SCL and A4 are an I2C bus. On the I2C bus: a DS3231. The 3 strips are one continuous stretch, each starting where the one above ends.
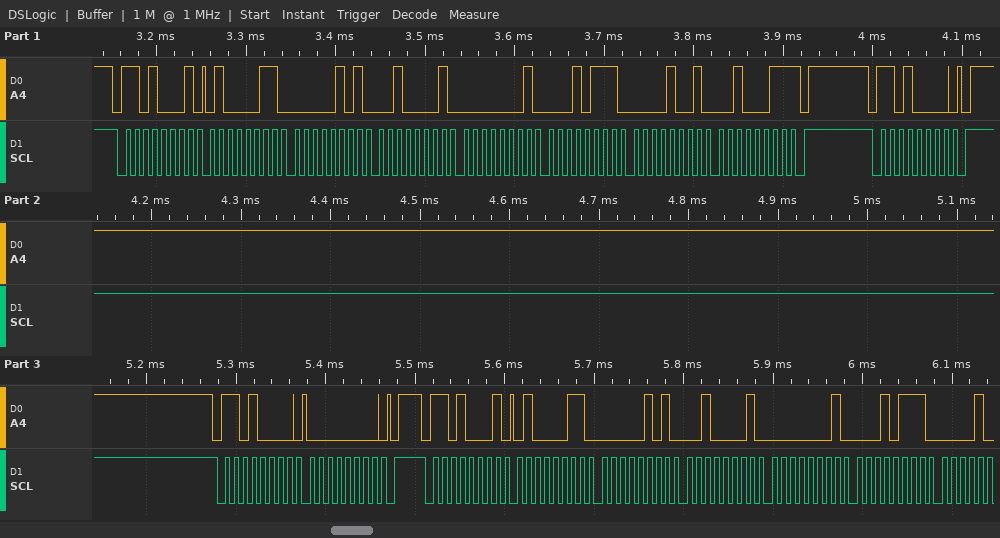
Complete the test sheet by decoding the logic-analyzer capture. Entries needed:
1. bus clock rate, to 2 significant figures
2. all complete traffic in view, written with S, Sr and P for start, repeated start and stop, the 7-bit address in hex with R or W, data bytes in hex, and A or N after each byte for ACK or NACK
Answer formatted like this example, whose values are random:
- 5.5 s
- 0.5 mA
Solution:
- 100 kHz
- S 68R A 43 A 05 A 21 A 01 A 17 A 09 A 23 N P S 68W A P S 68W A 00 A P S 68R A 43 A 05 A 21 A 01 A 17 A
